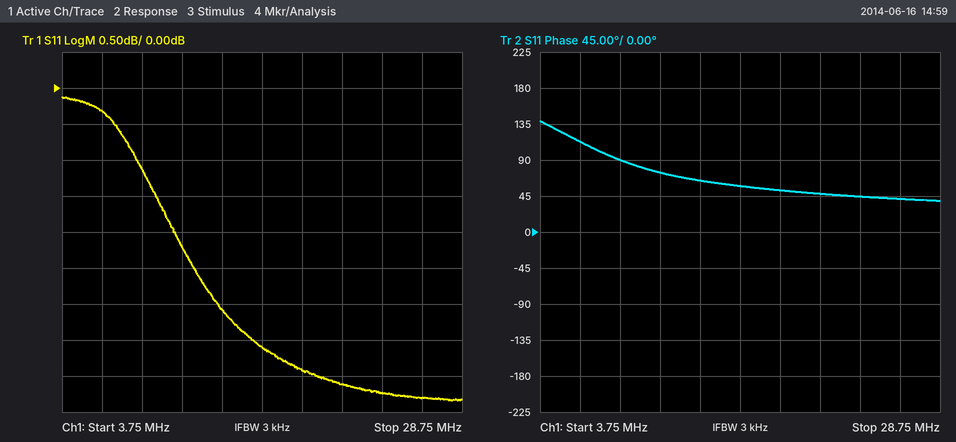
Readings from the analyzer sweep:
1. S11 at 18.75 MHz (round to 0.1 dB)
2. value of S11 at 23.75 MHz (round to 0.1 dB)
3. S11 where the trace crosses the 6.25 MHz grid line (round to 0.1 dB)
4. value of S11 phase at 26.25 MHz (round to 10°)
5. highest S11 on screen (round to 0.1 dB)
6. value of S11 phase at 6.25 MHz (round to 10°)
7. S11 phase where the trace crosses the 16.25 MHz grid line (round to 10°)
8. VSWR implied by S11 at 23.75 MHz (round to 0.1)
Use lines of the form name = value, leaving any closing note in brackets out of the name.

S11 at 18.75 MHz = -3.9 dB
value of S11 at 23.75 MHz = -4.2 dB
S11 where the trace crosses the 6.25 MHz grid line = -0.3 dB
value of S11 phase at 26.25 MHz = 40°
highest S11 on screen = -0.1 dB
value of S11 phase at 6.25 MHz = 110°
S11 phase where the trace crosses the 16.25 MHz grid line = 60°
VSWR implied by S11 at 23.75 MHz = 4.2
